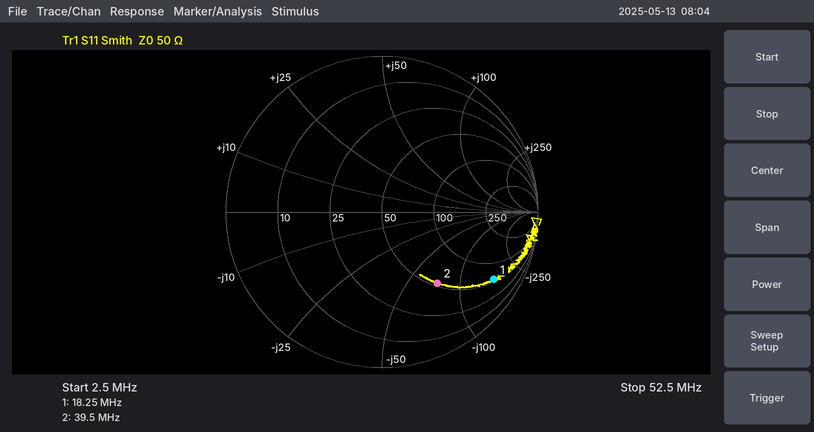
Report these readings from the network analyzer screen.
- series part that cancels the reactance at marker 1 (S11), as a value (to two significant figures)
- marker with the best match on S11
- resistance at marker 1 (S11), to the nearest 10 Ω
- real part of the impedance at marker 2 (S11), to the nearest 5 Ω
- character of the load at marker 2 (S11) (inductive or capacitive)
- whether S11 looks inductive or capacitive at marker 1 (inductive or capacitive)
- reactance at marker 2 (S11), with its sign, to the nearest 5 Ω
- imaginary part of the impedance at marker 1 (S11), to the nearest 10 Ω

1.4 µH
marker 2
60 Ω
55 Ω
capacitive
capacitive
-75 Ω
-160 Ω
